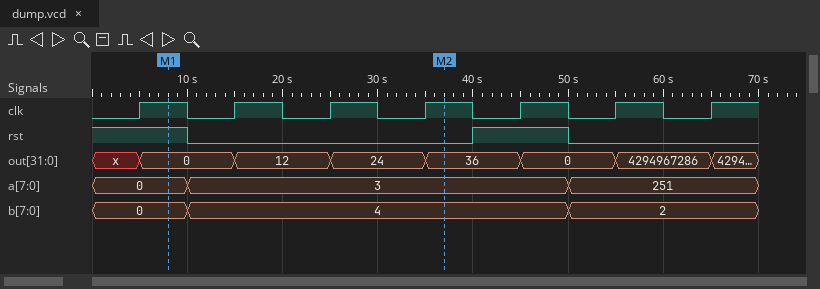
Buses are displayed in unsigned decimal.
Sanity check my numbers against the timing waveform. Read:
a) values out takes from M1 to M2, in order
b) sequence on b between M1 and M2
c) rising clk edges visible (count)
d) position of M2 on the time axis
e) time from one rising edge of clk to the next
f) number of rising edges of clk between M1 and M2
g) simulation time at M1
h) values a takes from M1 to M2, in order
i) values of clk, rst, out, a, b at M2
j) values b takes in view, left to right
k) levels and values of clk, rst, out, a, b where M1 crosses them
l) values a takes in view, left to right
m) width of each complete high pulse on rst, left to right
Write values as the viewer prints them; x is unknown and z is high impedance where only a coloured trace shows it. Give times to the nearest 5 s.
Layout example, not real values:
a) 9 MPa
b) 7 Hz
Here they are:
a) 0, 12, 24, 36
b) 0, 4
c) 7
d) 35 s
e) 10 s
f) 3
g) 10 s
h) 0, 3
i) clk=1, rst=0, out=36, a=3, b=4
j) 0, 4, 2
k) clk=1, rst=1, out=0, a=0, b=0
l) 0, 3, 251
m) 10 s
